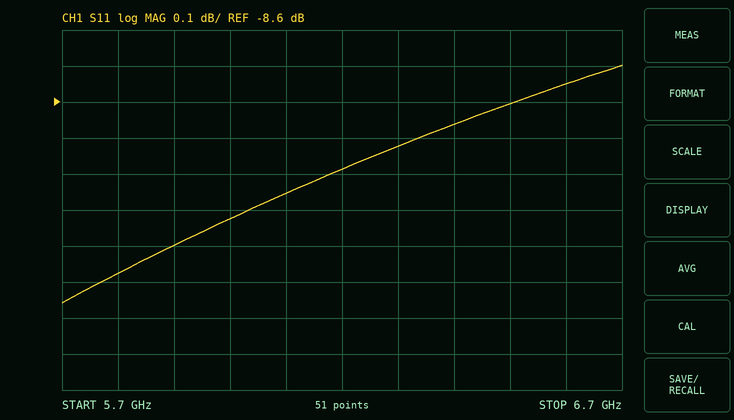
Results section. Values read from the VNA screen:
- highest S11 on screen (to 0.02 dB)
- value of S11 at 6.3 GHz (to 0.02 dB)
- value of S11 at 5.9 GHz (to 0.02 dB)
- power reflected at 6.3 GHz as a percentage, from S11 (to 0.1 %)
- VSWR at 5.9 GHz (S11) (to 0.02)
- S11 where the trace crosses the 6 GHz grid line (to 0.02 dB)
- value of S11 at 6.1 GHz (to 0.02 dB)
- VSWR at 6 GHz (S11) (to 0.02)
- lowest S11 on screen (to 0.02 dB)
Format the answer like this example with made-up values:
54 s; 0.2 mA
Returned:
-8.50 dB; -8.72 dB; -9.00 dB; 13.4 %; 2.10; -8.92 dB; -8.86 dB; 2.12; -9.16 dB
